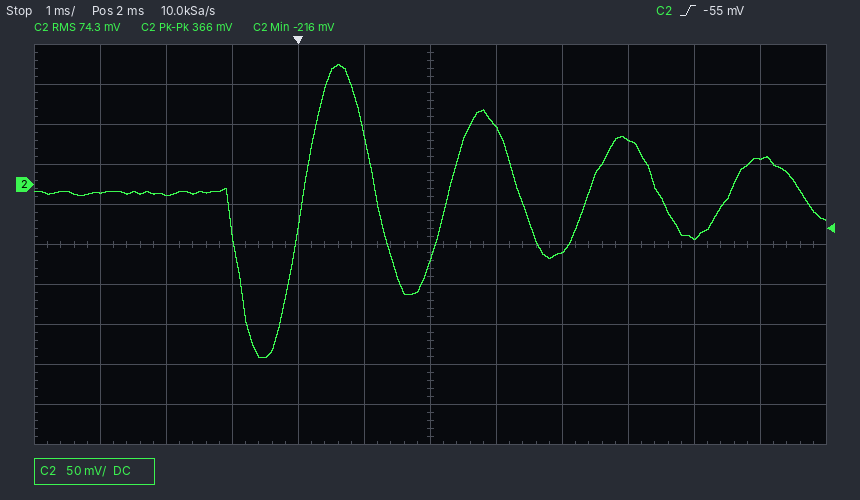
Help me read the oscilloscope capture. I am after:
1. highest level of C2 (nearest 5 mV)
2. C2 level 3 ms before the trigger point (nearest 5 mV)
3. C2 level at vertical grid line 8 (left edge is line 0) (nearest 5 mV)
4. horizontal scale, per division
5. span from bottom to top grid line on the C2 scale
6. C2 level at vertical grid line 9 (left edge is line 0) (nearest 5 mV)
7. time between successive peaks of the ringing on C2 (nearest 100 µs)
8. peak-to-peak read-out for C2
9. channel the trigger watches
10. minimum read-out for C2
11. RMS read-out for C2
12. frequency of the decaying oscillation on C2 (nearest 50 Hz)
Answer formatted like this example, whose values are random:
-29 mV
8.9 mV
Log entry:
150 mV
-10 mV
-85 mV
1 ms
500 mV
55 mV
2.2 ms
366 mV
C2
-216 mV
74.3 mV
450 Hz
